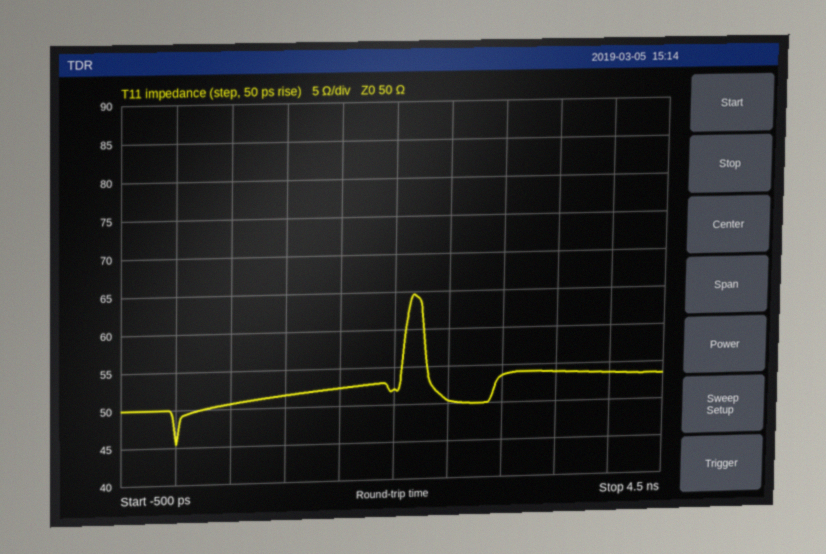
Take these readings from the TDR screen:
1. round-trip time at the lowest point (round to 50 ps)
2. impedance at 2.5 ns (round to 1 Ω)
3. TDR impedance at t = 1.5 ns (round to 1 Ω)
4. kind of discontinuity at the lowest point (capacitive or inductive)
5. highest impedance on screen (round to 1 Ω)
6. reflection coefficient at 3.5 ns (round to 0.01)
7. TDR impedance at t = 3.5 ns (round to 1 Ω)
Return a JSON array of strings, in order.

["0 ps", "50 Ω", "52 Ω", "capacitive", "65 Ω", "+0.04", "54 Ω"]
